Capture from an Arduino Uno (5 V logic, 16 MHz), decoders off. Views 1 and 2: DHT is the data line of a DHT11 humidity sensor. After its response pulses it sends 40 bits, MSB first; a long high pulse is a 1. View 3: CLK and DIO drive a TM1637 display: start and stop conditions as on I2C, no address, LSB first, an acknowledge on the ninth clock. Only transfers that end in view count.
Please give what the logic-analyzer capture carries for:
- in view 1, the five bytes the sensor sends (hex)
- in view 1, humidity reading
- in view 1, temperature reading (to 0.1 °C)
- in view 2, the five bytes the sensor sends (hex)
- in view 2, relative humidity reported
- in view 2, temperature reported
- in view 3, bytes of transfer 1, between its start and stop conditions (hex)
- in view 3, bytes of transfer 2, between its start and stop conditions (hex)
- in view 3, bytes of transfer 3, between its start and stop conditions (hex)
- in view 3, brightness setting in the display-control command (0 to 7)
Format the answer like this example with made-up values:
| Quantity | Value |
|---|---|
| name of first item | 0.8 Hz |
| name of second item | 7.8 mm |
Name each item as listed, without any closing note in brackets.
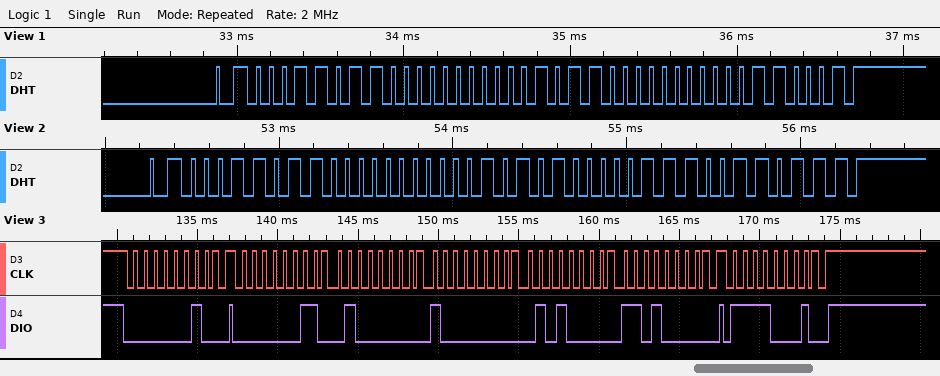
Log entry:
| Quantity | Value |
|---|---|
| in view 1, the five bytes the sensor sends | 1B 00 16 00 31 |
| in view 1, humidity reading | 27 % |
| in view 1, temperature reading | 22.0 °C |
| in view 2, the five bytes the sensor sends | 1B 00 15 07 37 |
| in view 2, relative humidity reported | 27 % |
| in view 2, temperature reported | 21.7 °C |
| in view 3, bytes of transfer 1, between its start and stop conditions | 40 |
| in view 3, bytes of transfer 2, between its start and stop conditions | C0 02 01 0A 0B |
| in view 3, bytes of transfer 3, between its start and stop conditions | 8F |
| in view 3, brightness setting in the display-control command | 7 |
